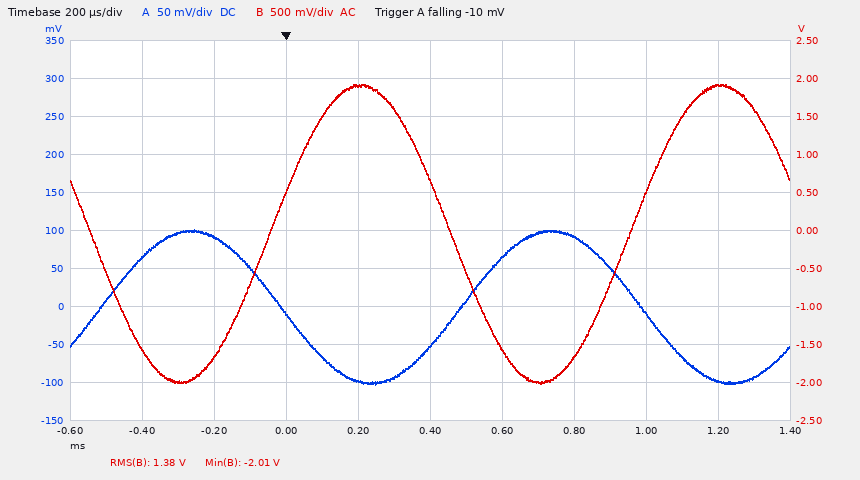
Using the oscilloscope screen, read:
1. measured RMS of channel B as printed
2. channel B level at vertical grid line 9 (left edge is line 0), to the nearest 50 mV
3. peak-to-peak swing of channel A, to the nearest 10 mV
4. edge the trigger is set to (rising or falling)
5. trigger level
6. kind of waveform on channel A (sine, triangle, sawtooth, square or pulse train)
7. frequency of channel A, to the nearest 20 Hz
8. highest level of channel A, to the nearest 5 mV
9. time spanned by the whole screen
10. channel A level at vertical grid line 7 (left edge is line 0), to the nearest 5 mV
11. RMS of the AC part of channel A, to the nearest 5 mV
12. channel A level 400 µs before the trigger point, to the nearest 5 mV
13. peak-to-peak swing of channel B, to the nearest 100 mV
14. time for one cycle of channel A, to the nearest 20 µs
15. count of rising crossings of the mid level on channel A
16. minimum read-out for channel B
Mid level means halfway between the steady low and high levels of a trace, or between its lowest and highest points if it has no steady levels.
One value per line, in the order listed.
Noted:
1.38 V
1.90 V
200 mV
falling
-10 mV
sine
1.00 kHz
100 mV
2 ms
90 mV
70 mV
65 mV
3.90 V
1.00 ms
2
-2.01 V
